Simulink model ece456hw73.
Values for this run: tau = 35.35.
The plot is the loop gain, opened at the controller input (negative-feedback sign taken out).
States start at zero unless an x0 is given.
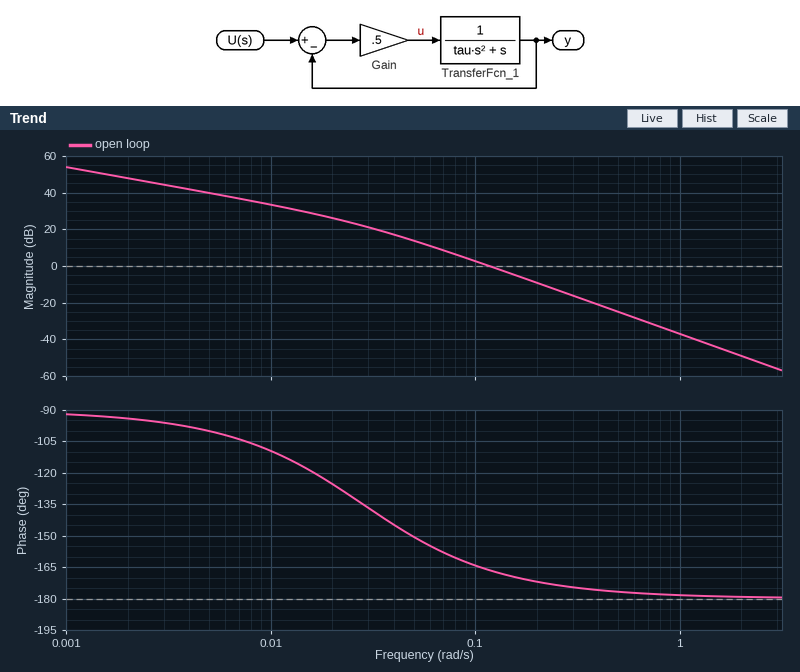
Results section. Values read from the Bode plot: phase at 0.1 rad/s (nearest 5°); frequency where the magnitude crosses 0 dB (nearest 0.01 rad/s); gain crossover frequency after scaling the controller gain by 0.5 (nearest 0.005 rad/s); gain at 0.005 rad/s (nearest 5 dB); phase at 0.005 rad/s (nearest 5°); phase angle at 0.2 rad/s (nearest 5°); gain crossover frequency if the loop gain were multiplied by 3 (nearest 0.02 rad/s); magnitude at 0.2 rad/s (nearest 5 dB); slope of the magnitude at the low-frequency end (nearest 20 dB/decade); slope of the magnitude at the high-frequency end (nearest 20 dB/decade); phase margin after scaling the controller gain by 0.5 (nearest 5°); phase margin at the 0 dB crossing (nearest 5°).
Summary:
-165°
0.12 rad/s
0.080 rad/s
40 dB
-100°
-170°
0.20 rad/s
-10 dB
-20 dB/decade
-40 dB/decade
20°
15°
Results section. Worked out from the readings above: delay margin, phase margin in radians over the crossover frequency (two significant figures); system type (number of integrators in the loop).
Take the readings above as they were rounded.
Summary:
2.2 s
1
